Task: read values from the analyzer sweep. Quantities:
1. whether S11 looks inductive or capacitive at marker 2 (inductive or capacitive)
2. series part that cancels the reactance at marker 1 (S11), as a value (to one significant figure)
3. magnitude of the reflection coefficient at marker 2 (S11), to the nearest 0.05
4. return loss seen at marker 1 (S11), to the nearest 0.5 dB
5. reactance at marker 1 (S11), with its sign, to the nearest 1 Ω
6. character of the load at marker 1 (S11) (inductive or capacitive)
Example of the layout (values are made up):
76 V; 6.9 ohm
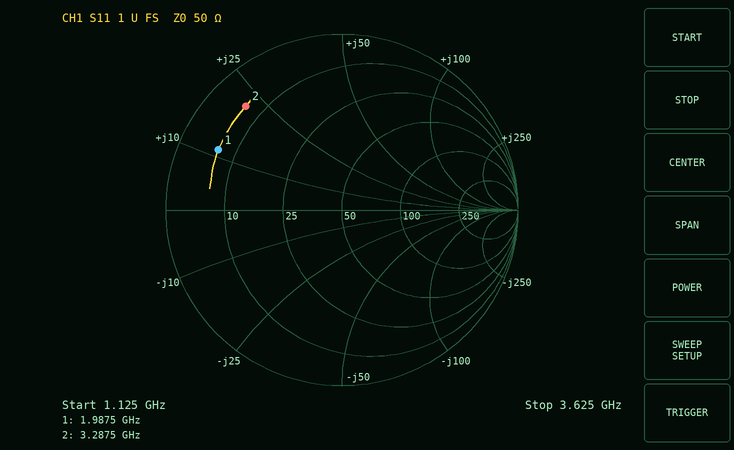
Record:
inductive; 7 pF; 0.80; 2.0 dB; +11 Ω; inductive
